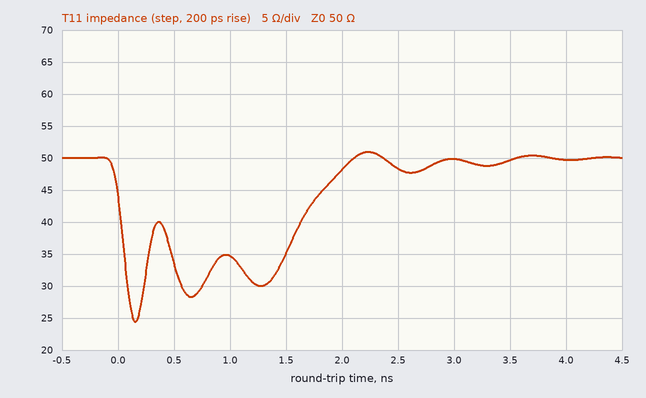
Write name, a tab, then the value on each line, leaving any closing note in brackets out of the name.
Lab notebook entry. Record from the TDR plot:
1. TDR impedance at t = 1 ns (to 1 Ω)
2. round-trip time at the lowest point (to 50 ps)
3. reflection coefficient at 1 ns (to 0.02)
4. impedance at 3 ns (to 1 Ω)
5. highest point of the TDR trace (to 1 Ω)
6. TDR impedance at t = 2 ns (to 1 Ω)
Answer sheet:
TDR impedance at t = 1 ns	35 Ω
round-trip time at the lowest point	150 ps
reflection coefficient at 1 ns	-0.18
impedance at 3 ns	50 Ω
highest point of the TDR trace	51 Ω
TDR impedance at t = 2 ns	48 Ω
